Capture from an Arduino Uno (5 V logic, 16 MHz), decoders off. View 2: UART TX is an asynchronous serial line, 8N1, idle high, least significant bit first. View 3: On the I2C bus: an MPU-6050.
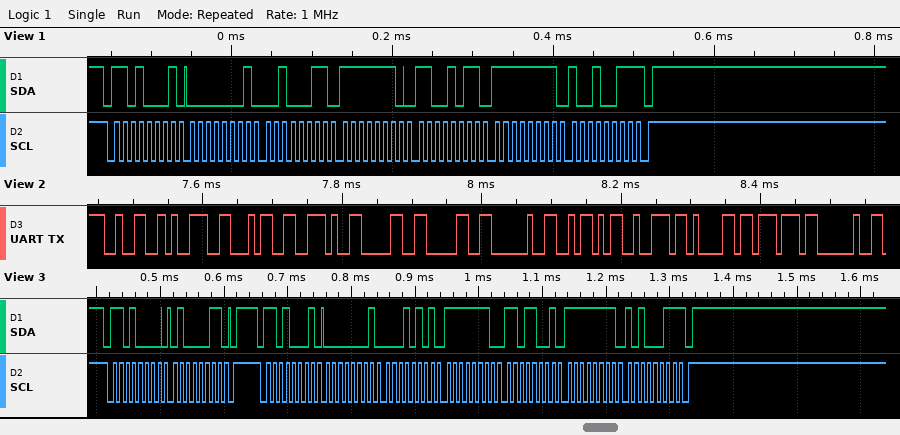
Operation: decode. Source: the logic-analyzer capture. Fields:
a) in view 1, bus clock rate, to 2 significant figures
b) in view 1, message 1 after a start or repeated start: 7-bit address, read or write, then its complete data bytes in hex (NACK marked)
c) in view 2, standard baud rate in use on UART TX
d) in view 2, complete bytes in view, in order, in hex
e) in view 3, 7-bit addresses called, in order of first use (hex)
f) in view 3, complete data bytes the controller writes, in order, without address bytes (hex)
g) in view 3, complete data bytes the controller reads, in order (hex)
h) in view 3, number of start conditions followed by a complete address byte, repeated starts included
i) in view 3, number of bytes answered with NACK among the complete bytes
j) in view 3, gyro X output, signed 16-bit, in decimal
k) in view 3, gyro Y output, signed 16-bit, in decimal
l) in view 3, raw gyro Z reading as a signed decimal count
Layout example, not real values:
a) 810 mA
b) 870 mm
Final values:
a) 100 kHz
b) 0x68 read: 01 23 FE CB FF 93 NACK
c) 115200 baud
d) 32 39 34 2E 30 30 20 5A 72 61 77 20
e) 0x68
f) 43
g) 01 15 FE D9 FF A3
h) 2
i) 1
j) 277
k) -295
l) -93
